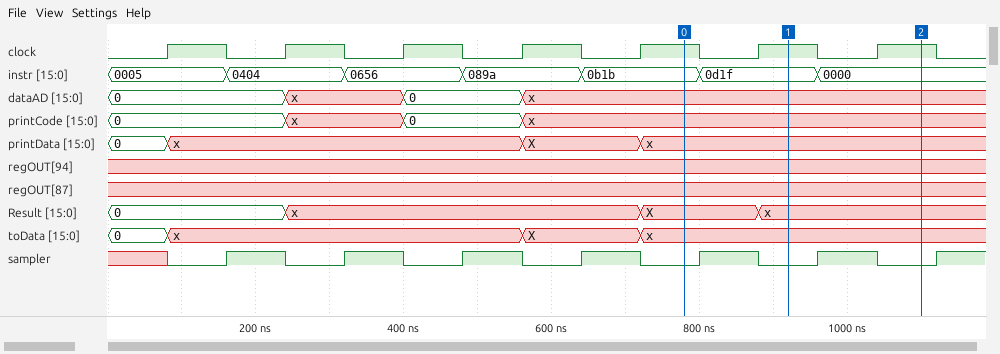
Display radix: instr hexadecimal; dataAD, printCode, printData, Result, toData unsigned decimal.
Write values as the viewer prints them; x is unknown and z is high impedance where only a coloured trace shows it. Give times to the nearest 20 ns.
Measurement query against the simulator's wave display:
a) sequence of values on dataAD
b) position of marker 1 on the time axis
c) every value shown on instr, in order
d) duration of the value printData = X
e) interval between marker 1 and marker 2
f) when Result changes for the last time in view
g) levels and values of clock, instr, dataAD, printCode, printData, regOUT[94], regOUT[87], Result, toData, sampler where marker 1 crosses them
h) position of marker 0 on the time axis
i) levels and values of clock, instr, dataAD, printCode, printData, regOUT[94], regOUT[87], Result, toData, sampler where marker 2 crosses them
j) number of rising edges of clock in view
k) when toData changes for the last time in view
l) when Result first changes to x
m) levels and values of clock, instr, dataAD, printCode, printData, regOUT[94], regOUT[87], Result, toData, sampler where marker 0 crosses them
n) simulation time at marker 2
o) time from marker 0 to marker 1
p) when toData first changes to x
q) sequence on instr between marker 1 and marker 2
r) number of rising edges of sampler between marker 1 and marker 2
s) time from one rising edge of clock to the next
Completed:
0, x, 0, x
920 ns
0005, 0404, 0656, 089a, 0b1b, 0d1f, 0000
160 ns
180 ns
880 ns
clock=1, instr=0d1f, dataAD=x, printCode=x, printData=x, regOUT[94]=x, regOUT[87]=x, Result=x, toData=x, sampler=0
780 ns
clock=1, instr=0000, dataAD=x, printCode=x, printData=x, regOUT[94]=x, regOUT[87]=x, Result=x, toData=x, sampler=0
7
720 ns
240 ns
clock=1, instr=0b1b, dataAD=x, printCode=x, printData=x, regOUT[94]=x, regOUT[87]=x, Result=X, toData=x, sampler=0
1100 ns
140 ns
80 ns
0d1f, 0000
1
160 ns
